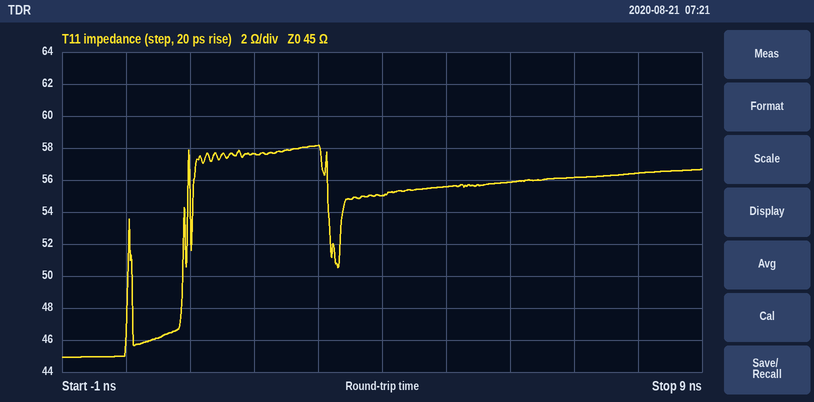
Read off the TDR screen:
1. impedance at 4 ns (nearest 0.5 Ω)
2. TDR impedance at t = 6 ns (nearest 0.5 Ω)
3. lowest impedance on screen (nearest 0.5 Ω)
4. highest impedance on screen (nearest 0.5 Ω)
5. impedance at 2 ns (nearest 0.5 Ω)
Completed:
55.0 Ω
56.0 Ω
45.0 Ω
58.0 Ω
57.5 Ω
